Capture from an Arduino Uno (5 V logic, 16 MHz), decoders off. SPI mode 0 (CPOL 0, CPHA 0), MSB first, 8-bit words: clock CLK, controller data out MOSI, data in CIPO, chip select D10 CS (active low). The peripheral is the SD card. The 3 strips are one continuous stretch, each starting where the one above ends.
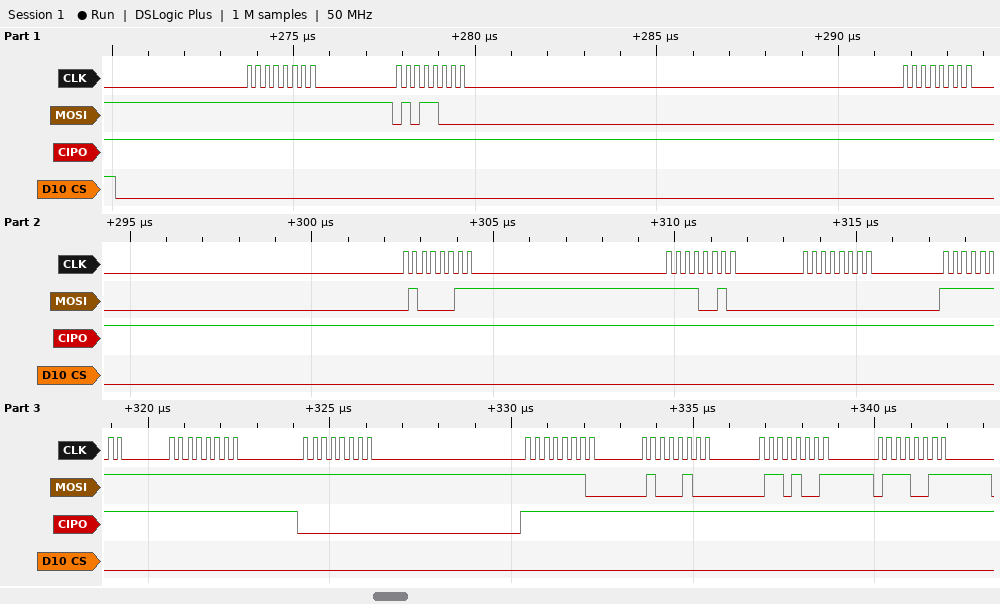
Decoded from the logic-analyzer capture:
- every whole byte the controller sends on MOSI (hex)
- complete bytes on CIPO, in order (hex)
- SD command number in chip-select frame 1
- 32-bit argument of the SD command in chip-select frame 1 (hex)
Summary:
0xFF 0x58 0x00 0x43 0xF2 0x00 0xFF 0xFF 0xFF 0xFE 0x44 0x69 0x73
0xFF 0xFF 0xFF 0xFF 0xFF 0xFF 0xFF 0xFF 0x00 0xFF 0xFF 0xFF 0xFF
CMD24
0x0043F200
